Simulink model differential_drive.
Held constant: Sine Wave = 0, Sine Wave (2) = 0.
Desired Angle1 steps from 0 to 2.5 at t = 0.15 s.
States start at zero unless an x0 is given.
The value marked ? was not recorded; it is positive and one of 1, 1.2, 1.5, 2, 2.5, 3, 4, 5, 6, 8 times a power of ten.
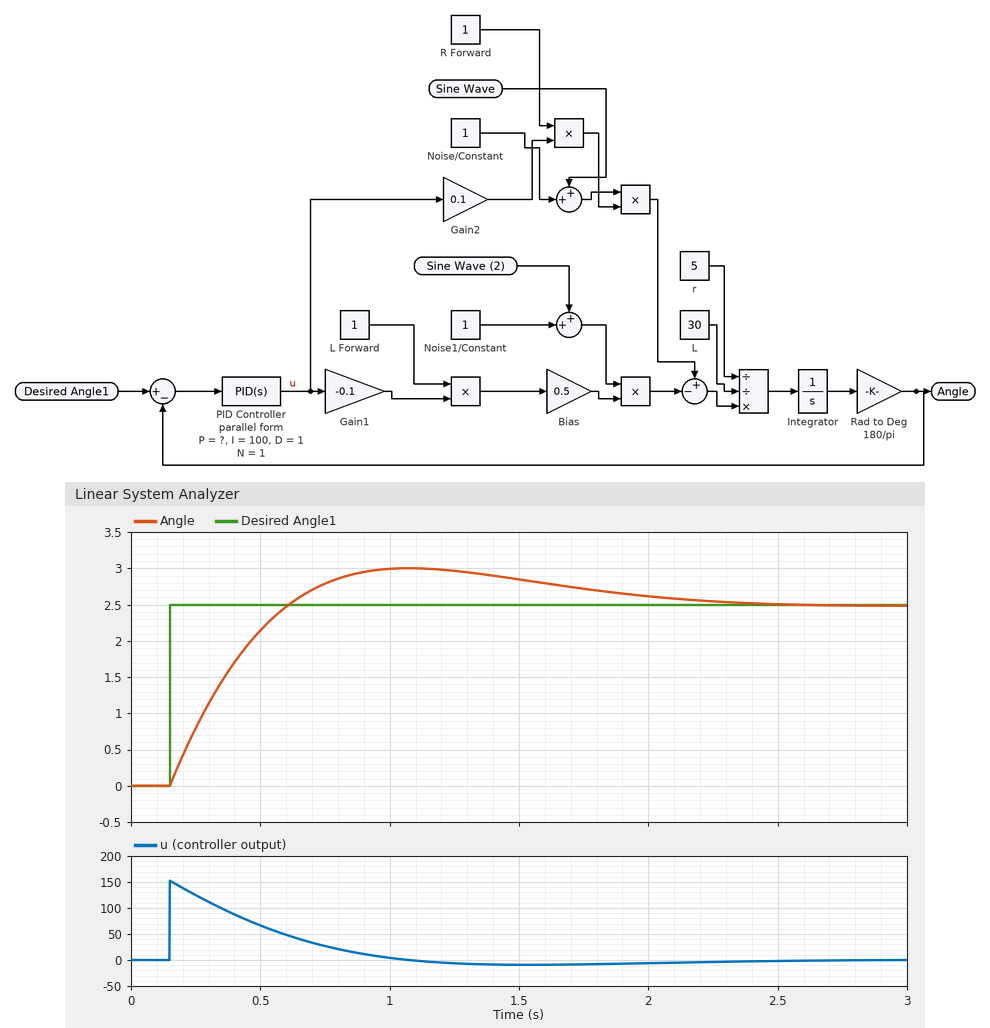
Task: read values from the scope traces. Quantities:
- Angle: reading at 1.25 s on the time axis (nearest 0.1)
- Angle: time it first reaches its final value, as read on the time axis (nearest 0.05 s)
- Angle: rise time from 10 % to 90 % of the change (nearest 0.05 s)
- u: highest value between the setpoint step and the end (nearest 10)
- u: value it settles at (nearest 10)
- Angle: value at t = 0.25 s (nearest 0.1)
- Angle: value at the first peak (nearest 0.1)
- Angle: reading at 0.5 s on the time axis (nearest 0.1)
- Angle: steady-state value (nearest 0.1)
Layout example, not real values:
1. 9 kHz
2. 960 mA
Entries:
1. 3.0
2. 0.60 s
3. 0.35 s
4. 150
5. 0
6. 0.8
7. 3.0
8. 2.1
9. 2.5
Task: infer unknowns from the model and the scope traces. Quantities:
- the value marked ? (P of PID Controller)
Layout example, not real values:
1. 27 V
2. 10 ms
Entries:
1. 60
